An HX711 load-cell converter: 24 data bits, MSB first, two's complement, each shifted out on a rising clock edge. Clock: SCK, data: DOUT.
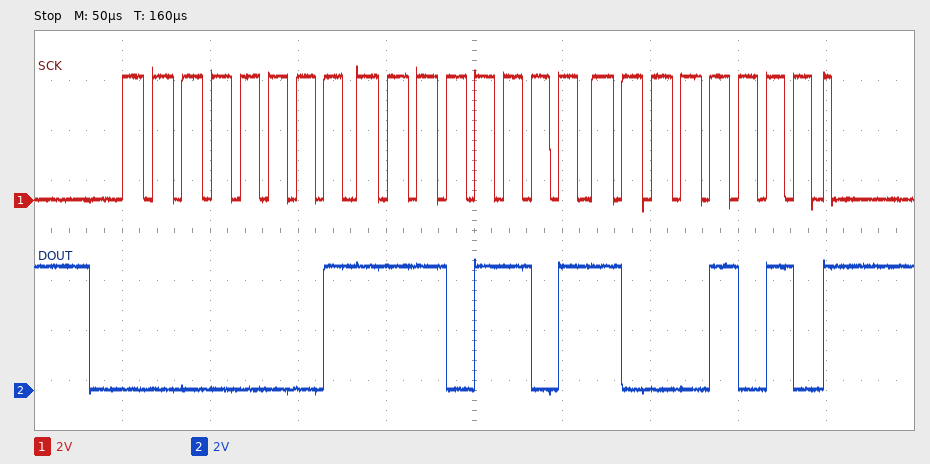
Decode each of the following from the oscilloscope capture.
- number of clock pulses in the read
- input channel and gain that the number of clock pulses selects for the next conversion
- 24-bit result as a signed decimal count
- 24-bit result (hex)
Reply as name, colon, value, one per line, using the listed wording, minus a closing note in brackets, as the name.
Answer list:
number of clock pulses in the read: 25
input channel and gain that the number of clock pulses selects for the next conversion: channel A, gain 128
24-bit result as a signed decimal count: 126346
24-bit result: 0x01ED8A
